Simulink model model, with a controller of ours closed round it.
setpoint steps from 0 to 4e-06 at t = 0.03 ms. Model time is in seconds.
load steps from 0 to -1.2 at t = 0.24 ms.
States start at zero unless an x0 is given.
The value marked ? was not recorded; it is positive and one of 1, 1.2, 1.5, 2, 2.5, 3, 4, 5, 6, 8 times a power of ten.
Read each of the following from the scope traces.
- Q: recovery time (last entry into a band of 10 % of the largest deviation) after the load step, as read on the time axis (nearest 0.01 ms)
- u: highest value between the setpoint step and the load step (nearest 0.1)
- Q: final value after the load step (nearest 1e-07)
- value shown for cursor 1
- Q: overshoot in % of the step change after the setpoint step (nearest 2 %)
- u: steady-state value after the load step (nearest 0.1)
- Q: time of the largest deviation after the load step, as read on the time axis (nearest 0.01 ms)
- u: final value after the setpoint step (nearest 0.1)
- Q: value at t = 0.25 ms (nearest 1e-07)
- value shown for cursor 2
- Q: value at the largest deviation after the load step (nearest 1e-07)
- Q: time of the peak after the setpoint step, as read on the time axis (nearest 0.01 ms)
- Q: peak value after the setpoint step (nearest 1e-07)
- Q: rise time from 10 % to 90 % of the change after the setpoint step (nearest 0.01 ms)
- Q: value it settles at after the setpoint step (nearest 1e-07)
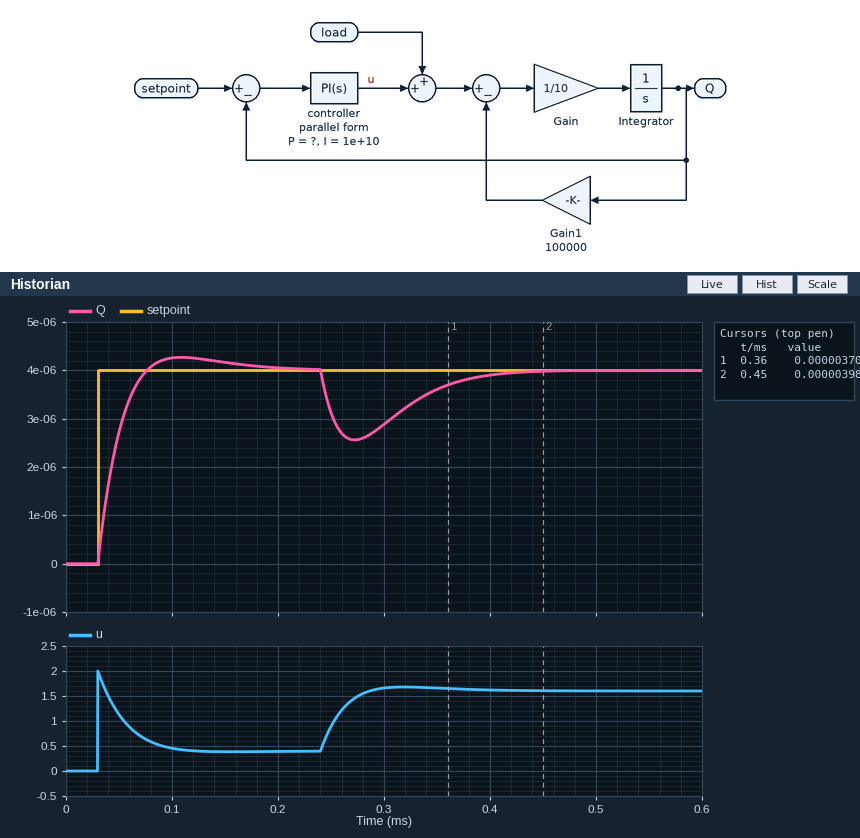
0.39 ms
2.0
0.0000040
0.00000370
6 %
1.6
0.27 ms
0.4
0.0000031
0.00000398
0.0000026
0.11 ms
0.0000043
0.03 ms
0.0000040
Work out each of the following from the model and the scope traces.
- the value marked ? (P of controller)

500000
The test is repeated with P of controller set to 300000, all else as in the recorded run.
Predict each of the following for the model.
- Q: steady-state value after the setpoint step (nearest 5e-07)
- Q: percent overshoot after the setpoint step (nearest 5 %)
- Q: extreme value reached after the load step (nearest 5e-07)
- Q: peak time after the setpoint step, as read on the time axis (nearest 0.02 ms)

0.0000040
15 %
0.0000020
0.12 ms
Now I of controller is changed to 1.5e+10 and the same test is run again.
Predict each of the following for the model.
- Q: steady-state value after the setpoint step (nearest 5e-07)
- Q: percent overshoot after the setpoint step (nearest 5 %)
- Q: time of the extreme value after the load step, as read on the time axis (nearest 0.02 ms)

0.0000040
10 %
0.26 ms
